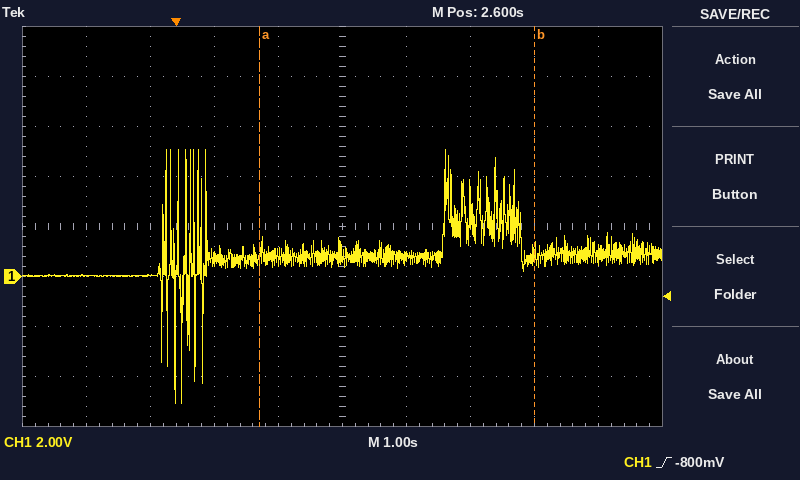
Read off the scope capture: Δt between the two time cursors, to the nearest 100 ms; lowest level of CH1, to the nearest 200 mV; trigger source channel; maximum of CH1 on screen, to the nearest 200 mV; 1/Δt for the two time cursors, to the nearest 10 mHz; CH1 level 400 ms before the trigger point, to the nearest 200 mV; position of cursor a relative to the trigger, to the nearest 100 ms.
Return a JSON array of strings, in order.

["4.3 s", "-5.0 V", "CH1", "5.0 V", "230 mHz", "0.0 V", "+1.3 s"]
